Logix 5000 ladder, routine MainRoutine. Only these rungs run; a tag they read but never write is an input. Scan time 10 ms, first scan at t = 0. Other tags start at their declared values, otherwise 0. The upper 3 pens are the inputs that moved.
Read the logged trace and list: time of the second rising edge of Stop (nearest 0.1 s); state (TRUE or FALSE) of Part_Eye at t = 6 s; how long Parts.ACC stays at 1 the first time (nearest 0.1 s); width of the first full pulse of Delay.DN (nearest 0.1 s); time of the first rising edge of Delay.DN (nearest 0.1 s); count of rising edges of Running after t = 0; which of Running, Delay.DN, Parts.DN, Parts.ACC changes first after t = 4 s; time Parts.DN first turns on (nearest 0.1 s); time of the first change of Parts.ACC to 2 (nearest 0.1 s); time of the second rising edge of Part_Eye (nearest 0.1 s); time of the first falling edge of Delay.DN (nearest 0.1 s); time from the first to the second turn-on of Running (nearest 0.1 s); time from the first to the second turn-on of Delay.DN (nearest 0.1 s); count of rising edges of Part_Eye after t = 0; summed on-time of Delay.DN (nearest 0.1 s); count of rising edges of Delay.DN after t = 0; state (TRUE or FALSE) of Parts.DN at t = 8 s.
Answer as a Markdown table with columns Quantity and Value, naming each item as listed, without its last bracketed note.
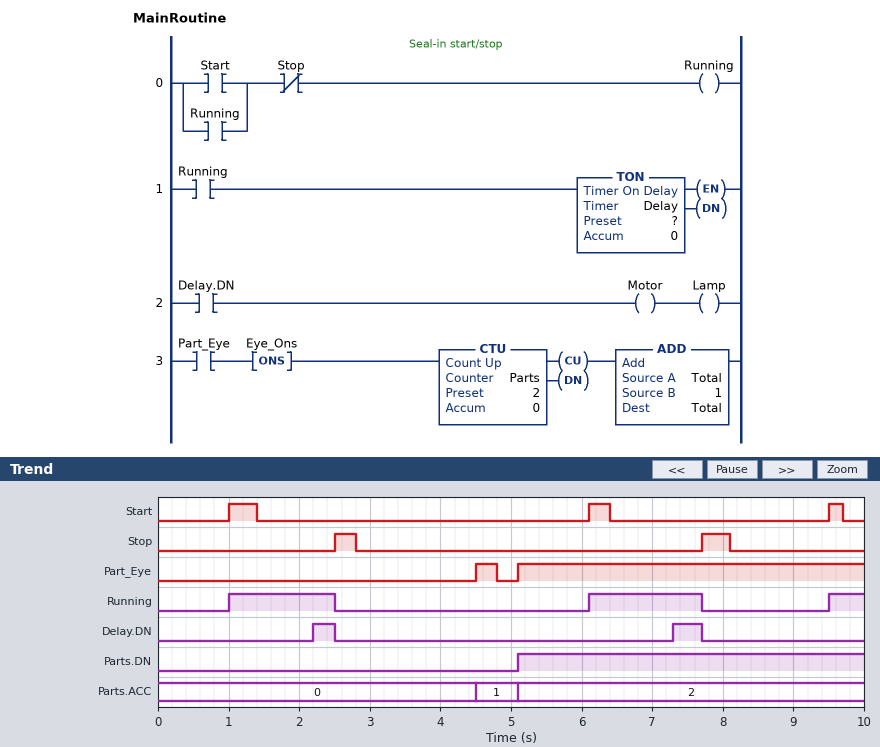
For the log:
| Quantity | Value |
|---|---|
| time of the second rising edge of Stop | 7.7 s |
| state (TRUE or FALSE) of Part_Eye at t = 6 s | TRUE |
| how long Parts.ACC stays at 1 the first time | 0.6 s |
| width of the first full pulse of Delay.DN | 0.3 s |
| time of the first rising edge of Delay.DN | 2.2 s |
| count of rising edges of Running after t = 0 | 3 |
| which of Running, Delay.DN, Parts.DN, Parts.ACC changes first after t = 4 s | Parts.ACC |
| time Parts.DN first turns on | 5.1 s |
| time of the first change of Parts.ACC to 2 | 5.1 s |
| time of the second rising edge of Part_Eye | 5.1 s |
| time of the first falling edge of Delay.DN | 2.5 s |
| time from the first to the second turn-on of Running | 5.1 s |
| time from the first to the second turn-on of Delay.DN | 5.1 s |
| count of rising edges of Part_Eye after t = 0 | 2 |
| summed on-time of Delay.DN | 0.7 s |
| count of rising edges of Delay.DN after t = 0 | 2 |
| state (TRUE or FALSE) of Parts.DN at t = 8 s | TRUE |
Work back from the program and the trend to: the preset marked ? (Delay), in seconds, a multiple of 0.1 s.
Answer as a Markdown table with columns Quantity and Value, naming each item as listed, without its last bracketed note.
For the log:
| Quantity | Value |
|---|---|
| the preset marked ? (Delay), in seconds, a multiple of 0.1 s | 1.2 s |
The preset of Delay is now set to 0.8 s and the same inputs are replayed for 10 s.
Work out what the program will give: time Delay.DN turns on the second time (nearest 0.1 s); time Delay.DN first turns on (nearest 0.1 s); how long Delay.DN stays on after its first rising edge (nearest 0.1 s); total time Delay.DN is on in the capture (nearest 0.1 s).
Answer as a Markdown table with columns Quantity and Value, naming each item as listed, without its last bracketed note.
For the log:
| Quantity | Value |
|---|---|
| time Delay.DN turns on the second time | 6.9 s |
| time Delay.DN first turns on | 1.8 s |
| how long Delay.DN stays on after its first rising edge | 0.7 s |
| total time Delay.DN is on in the capture | 1.5 s |
